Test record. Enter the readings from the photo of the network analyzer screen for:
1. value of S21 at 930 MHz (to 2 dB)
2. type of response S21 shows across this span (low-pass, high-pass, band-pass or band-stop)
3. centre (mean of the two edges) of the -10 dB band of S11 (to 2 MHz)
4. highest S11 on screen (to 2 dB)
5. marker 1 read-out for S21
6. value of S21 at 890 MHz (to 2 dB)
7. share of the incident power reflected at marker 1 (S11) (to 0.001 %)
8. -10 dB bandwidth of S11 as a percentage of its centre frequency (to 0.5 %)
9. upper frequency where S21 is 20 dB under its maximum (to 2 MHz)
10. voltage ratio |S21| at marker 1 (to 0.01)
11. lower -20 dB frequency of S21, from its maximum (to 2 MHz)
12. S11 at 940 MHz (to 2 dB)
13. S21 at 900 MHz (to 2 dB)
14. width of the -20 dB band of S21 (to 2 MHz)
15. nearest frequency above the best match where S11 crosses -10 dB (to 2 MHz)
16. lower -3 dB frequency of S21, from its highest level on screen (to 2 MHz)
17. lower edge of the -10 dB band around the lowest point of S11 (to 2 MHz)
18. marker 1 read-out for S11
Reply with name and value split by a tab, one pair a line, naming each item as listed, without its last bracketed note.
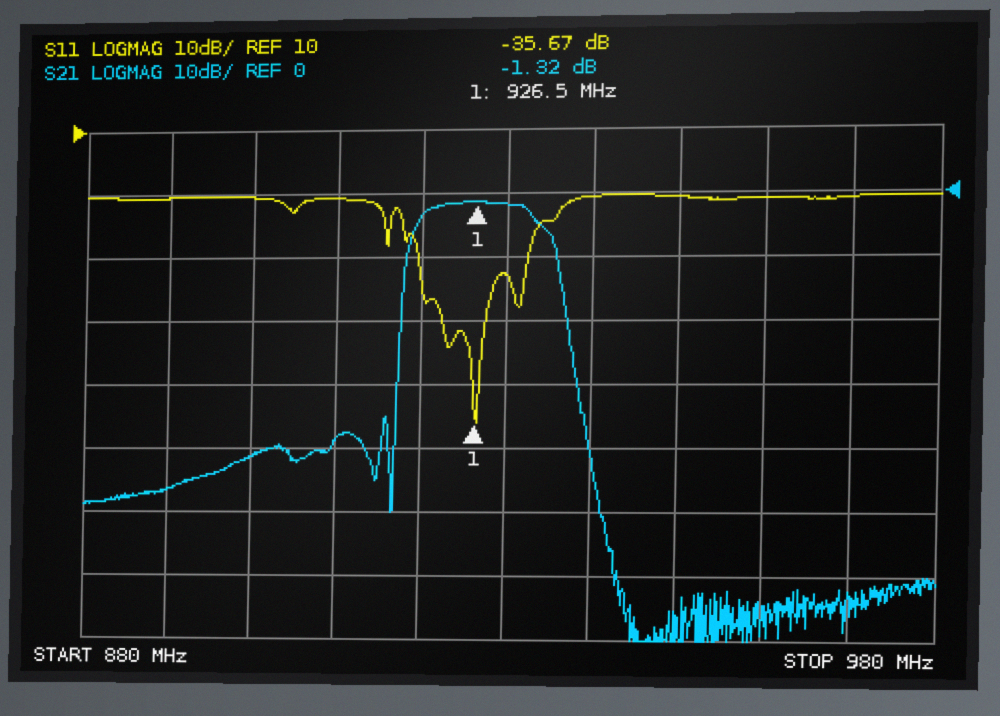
value of S21 at 930 MHz	-2 dB
type of response S21 shows across this span	band-pass
centre (mean of the two edges) of the -10 dB band of S11	926 MHz
highest S11 on screen	0 dB
marker 1 read-out for S21	-1.32 dB
value of S21 at 890 MHz	-46 dB
share of the incident power reflected at marker 1 (S11)	0.027 %
-10 dB bandwidth of S11 as a percentage of its centre frequency	1.5 %
upper frequency where S21 is 20 dB under its maximum	938 MHz
voltage ratio |S21| at marker 1	0.86
lower -20 dB frequency of S21, from its maximum	918 MHz
S11 at 940 MHz	0 dB
S21 at 900 MHz	-42 dB
width of the -20 dB band of S21	20 MHz
nearest frequency above the best match where S11 crosses -10 dB	932 MHz
lower -3 dB frequency of S21, from its highest level on screen	920 MHz
lower edge of the -10 dB band around the lowest point of S11	920 MHz
marker 1 read-out for S11	-35.67 dB
